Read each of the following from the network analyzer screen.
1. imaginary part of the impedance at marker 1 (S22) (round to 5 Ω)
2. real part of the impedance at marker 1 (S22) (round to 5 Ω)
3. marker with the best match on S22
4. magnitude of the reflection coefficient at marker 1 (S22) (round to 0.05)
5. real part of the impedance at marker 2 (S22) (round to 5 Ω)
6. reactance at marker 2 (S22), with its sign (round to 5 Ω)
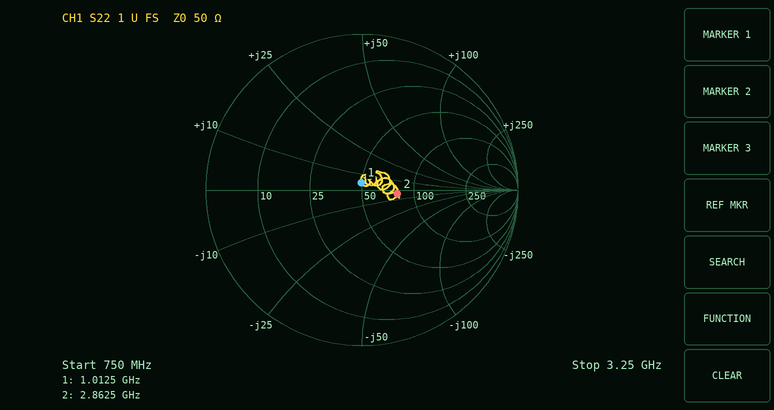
+5 Ω
50 Ω
marker 1
0.05
80 Ω
-5 Ω
